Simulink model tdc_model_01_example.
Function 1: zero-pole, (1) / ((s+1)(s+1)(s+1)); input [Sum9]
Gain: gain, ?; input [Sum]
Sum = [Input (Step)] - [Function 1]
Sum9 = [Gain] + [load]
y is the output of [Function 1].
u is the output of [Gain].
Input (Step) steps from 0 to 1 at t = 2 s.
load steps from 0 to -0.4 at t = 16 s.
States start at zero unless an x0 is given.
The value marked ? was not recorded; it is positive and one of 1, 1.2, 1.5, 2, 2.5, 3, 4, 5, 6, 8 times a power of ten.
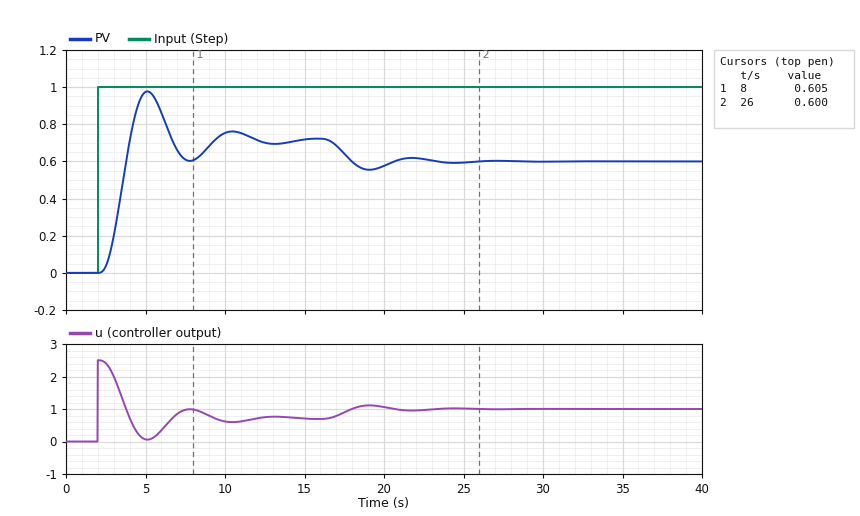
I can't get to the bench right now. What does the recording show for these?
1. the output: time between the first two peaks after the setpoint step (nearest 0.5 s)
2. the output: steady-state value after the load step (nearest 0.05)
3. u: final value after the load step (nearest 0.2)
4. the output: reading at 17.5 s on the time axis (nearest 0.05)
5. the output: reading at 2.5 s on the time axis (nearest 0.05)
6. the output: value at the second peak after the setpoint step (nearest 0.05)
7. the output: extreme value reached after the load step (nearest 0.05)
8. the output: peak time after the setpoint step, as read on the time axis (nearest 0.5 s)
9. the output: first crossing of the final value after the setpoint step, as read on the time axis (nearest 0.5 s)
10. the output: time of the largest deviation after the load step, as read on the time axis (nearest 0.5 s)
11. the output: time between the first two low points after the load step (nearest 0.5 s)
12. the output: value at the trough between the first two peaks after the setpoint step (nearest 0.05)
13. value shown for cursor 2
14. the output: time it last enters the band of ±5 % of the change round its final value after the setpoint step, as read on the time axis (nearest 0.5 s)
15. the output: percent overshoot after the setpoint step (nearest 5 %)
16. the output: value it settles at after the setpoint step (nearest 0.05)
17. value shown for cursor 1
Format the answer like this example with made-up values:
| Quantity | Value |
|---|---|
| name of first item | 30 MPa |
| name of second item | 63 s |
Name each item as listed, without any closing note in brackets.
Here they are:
| Quantity | Value |
|---|---|
| the output: time between the first two peaks after the setpoint step | 5.5 s |
| the output: steady-state value after the load step | 0.60 |
| u: final value after the load step | 1.0 |
| the output: reading at 17.5 s on the time axis | 0.65 |
| the output: reading at 2.5 s on the time axis | 0.05 |
| the output: value at the second peak after the setpoint step | 0.75 |
| the output: extreme value reached after the load step | 0.55 |
| the output: peak time after the setpoint step, as read on the time axis | 5.0 s |
| the output: first crossing of the final value after the setpoint step, as read on the time axis | 4.0 s |
| the output: time of the largest deviation after the load step, as read on the time axis | 19.0 s |
| the output: time between the first two low points after the load step | 5.5 s |
| the output: value at the trough between the first two peaks after the setpoint step | 0.60 |
| value shown for cursor 2 | 0.600 |
| the output: time it last enters the band of ±5 % of the change round its final value after the setpoint step, as read on the time axis | 11.0 s |
| the output: percent overshoot after the setpoint step | 35 % |
| the output: value it settles at after the setpoint step | 0.70 |
| value shown for cursor 1 | 0.605 |
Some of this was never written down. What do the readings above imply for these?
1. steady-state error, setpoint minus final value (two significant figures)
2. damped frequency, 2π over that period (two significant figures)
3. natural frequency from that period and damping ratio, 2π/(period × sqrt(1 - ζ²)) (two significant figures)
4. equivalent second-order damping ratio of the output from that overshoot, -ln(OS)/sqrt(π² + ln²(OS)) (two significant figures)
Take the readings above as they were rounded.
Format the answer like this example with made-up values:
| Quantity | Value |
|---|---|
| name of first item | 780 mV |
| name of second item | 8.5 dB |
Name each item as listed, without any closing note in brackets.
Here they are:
| Quantity | Value |
|---|---|
| steady-state error, setpoint minus final value | 0.30 |
| damped frequency, 2π over that period | 1.1 rad/s |
| natural frequency from that period and damping ratio, 2π/(period × sqrt(1 - ζ²)) | 1.2 rad/s |
| equivalent second-order damping ratio of the output from that overshoot, -ln(OS)/sqrt(π² + ln²(OS)) | 0.32 |
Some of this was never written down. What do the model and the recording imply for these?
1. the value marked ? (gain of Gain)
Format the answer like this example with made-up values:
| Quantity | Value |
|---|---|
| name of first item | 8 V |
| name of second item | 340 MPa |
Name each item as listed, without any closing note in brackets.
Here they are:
| Quantity | Value |
|---|---|
| the value marked ? | 2.5 |
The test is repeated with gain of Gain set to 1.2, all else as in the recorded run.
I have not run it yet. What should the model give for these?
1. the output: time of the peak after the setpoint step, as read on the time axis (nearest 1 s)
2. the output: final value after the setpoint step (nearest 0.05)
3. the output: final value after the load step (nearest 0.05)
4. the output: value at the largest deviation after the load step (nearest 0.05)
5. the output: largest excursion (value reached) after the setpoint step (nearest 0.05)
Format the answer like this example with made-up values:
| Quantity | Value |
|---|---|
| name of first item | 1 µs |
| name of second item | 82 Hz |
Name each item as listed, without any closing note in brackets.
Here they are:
| Quantity | Value |
|---|---|
| the output: time of the peak after the setpoint step, as read on the time axis | 6 s |
| the output: final value after the setpoint step | 0.55 |
| the output: final value after the load step | 0.35 |
| the output: value at the largest deviation after the load step | 0.35 |
| the output: largest excursion (value reached) after the setpoint step | 0.65 |
